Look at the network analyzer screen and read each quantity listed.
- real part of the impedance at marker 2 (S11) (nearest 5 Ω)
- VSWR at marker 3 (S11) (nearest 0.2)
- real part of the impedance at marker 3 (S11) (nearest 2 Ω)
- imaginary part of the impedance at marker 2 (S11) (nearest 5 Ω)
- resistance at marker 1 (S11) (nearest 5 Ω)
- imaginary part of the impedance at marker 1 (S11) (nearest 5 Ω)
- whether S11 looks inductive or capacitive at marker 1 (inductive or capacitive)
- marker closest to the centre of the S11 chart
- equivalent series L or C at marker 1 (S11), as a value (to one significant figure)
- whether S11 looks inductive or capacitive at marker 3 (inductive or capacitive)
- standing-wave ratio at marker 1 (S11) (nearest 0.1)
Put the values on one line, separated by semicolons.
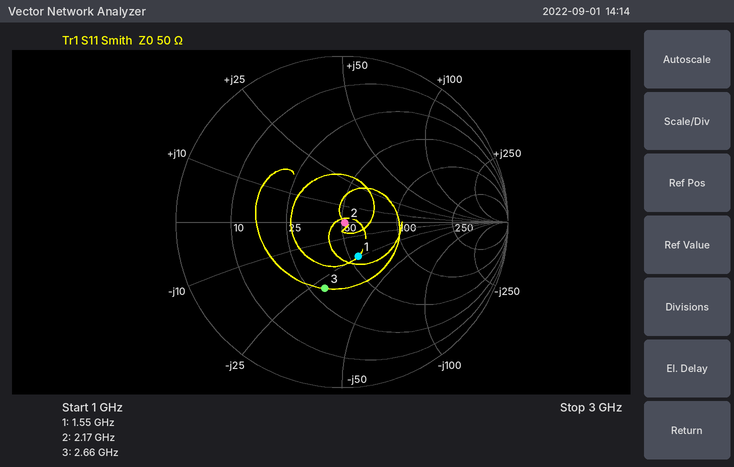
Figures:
50 Ω; 2.4; 30 Ω; 0 Ω; 55 Ω; -25 Ω; capacitive; marker 2; 4 pF; capacitive; 1.6
